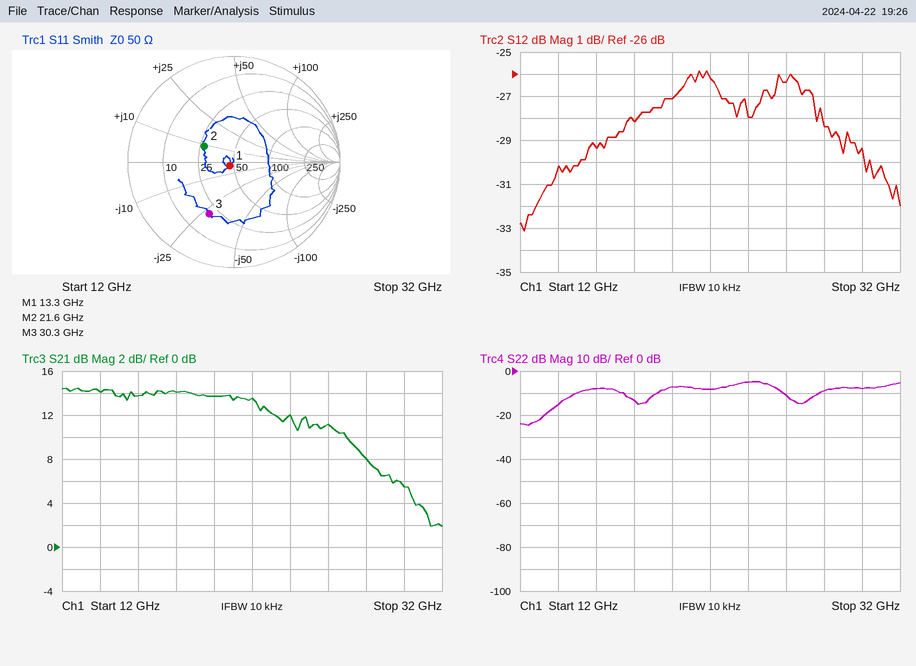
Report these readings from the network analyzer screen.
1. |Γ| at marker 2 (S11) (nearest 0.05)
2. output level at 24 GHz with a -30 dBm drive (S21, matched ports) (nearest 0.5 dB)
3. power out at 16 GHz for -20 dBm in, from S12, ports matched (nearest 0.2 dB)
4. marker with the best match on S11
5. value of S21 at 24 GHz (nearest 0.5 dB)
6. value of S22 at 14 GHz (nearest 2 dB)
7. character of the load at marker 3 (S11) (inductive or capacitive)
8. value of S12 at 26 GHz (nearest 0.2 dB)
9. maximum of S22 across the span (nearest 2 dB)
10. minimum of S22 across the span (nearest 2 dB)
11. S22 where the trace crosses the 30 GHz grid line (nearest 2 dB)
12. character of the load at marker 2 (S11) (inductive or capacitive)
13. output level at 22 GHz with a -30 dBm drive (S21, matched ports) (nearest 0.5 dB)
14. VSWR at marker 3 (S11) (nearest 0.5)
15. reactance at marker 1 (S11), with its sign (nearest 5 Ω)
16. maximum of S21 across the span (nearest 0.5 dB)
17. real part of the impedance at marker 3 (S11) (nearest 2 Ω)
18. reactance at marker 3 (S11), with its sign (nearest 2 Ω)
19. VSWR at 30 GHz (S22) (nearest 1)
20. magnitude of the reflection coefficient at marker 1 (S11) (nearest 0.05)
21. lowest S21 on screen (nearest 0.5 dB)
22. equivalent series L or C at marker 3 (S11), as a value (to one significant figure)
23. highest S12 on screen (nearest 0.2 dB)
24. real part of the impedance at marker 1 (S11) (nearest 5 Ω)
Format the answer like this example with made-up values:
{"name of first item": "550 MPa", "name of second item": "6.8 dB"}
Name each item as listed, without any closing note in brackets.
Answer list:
{"|Γ| at marker 2 (S11)": "0.30", "output level at 24 GHz with a -30 dBm drive (S21, matched ports)": "-18.0 dBm", "power out at 16 GHz for -20 dBm in, from S12, ports matched": "-49.4 dBm", "marker with the best match on S11": "marker 1", "value of S21 at 24 GHz": "12.0 dB", "value of S22 at 14 GHz": "-16 dB", "character of the load at marker 3 (S11)": "capacitive", "value of S12 at 26 GHz": "-26.4 dB", "maximum of S22 across the span": "-4 dB", "minimum of S22 across the span": "-24 dB", "S22 where the trace crosses the 30 GHz grid line": "-8 dB", "character of the load at marker 2 (S11)": "inductive", "output level at 22 GHz with a -30 dBm drive (S21, matched ports)": "-16.5 dBm", "VSWR at marker 3 (S11)": "3.5", "reactance at marker 1 (S11), with its sign": "-5 Ω", "maximum of S21 across the span": "14.5 dB", "real part of the impedance at marker 3 (S11)": "20 Ω", "reactance at marker 3 (S11), with its sign": "-28 Ω", "VSWR at 30 GHz (S22)": "2", "magnitude of the reflection coefficient at marker 1 (S11)": "0.05", "lowest S21 on screen": "2.0 dB", "equivalent series L or C at marker 3 (S11), as a value": "200 fF", "highest S12 on screen": "-25.8 dB", "real part of the impedance at marker 1 (S11)": "45 Ω"}
